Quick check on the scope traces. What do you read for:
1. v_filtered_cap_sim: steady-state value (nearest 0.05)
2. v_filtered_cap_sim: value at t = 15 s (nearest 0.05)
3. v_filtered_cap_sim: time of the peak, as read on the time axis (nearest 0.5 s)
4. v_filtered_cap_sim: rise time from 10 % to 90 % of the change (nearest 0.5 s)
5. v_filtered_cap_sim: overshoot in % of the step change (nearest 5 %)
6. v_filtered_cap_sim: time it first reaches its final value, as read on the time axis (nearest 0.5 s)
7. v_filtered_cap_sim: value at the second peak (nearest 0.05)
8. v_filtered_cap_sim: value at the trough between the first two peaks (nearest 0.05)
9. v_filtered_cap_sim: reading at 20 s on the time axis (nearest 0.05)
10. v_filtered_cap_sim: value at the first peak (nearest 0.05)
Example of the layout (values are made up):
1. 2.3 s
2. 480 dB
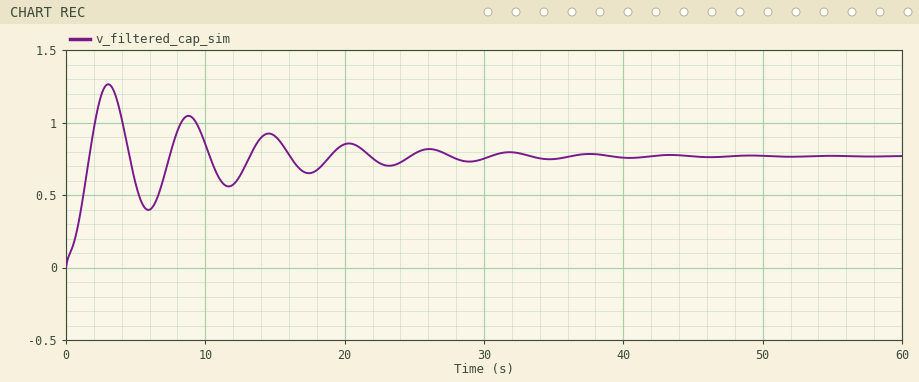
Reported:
1. 0.75
2. 0.90
3. 3.0 s
4. 1.5 s
5. 65 %
6. 1.5 s
7. 1.05
8. 0.40
9. 0.85
10. 1.25
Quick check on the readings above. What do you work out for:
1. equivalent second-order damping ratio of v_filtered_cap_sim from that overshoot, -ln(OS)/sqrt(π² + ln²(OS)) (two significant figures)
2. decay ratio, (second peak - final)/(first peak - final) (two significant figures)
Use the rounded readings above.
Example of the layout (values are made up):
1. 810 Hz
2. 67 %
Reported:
1. 0.14
2. 0.60
